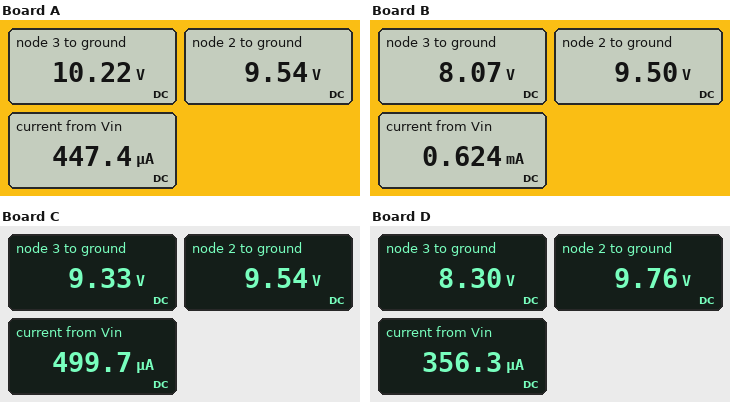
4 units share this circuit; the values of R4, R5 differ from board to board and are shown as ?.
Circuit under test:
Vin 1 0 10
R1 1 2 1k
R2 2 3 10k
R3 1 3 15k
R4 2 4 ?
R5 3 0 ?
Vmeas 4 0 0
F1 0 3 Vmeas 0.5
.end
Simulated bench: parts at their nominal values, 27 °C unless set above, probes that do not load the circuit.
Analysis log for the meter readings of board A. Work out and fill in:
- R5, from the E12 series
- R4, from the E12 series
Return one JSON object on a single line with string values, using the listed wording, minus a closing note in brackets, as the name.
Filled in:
{"R5, from the E12 series": "56 kΩ", "R4, from the E12 series": "18 kΩ"}
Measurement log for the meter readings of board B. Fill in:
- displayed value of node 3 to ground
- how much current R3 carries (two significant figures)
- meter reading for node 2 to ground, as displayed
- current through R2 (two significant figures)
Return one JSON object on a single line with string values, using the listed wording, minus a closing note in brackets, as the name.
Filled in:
{"displayed value of node 3 to ground": "8.07 V", "how much current R3 carries": "130 µA", "meter reading for node 2 to ground, as displayed": "9.50 V", "current through R2": "140 µA"}
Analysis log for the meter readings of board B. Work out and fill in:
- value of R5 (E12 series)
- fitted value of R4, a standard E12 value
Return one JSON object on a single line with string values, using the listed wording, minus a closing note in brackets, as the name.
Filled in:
{"value of R5": "18 kΩ", "fitted value of R4, a standard E12 value": "27 kΩ"}
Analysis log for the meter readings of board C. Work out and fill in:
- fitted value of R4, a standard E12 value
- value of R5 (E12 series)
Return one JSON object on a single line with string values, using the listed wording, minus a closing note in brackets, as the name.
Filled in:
{"fitted value of R4, a standard E12 value": "22 kΩ", "value of R5": "33 kΩ"}
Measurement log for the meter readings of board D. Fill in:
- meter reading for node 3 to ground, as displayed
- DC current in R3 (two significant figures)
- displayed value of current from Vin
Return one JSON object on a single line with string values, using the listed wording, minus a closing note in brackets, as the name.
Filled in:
{"meter reading for node 3 to ground, as displayed": "8.30 V", "DC current in R3": "110 µA", "displayed value of current from Vin": "356.3 µA"}
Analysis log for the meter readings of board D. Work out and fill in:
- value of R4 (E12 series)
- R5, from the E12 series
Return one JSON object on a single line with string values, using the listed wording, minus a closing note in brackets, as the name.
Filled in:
{"value of R4": "100 kΩ", "R5, from the E12 series": "27 kΩ"}
